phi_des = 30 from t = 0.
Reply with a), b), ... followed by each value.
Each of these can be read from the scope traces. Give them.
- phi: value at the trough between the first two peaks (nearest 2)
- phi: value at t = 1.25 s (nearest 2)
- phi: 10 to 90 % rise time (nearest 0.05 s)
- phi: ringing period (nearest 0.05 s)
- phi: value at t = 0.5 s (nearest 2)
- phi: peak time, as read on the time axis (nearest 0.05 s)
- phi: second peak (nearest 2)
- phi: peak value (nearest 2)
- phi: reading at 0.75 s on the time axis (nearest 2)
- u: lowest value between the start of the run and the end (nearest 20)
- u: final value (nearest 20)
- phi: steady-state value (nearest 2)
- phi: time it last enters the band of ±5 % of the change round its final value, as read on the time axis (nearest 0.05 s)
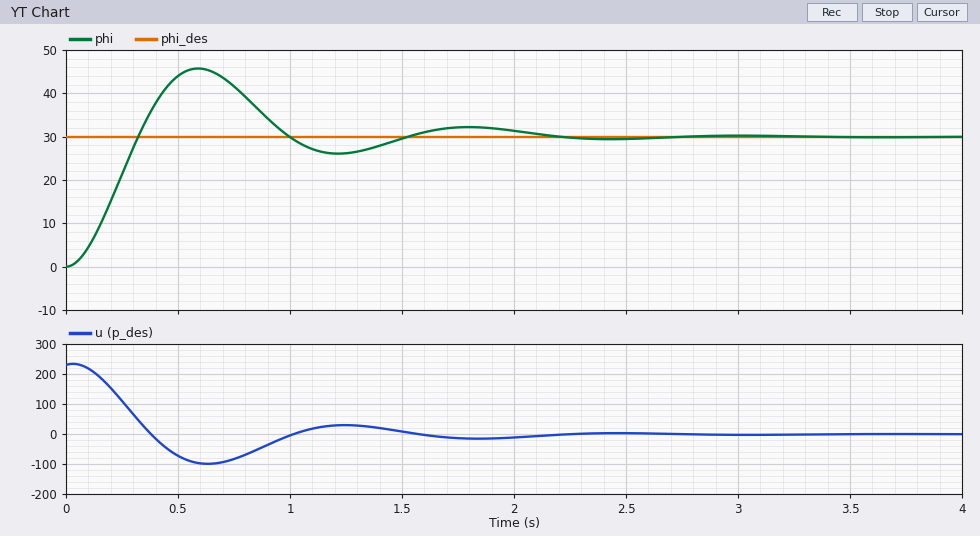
a) 26
b) 26
c) 0.20 s
d) 1.20 s
e) 44
f) 0.60 s
g) 32
h) 46
i) 42
j) -100
k) 0
l) 30
m) 2.00 s
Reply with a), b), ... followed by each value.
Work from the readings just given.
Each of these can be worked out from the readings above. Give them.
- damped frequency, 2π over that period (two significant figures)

a) 5.2 rad/s
